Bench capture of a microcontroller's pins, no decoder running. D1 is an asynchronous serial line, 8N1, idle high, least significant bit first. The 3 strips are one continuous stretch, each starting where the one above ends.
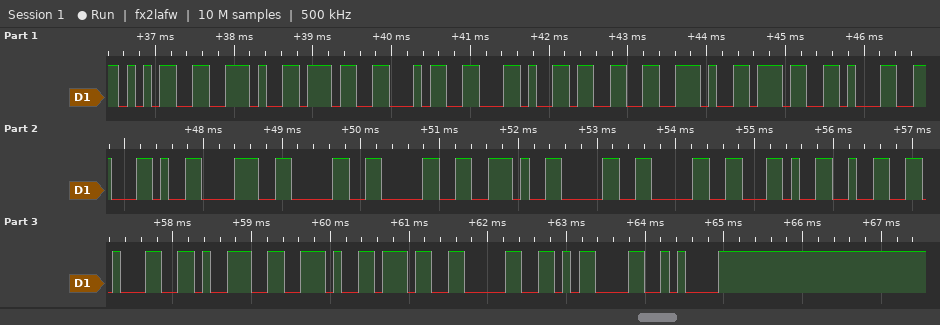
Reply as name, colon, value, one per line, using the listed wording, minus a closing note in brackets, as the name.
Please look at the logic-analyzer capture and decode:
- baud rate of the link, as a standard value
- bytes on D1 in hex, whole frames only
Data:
baud rate of the link, as a standard value: 9600 baud
bytes on D1 in hex, whole frames only: 0x35 0x2E 0x37 0x34 0x2C 0x33 0x2E 0x37 0x31 0x2C 0x38 0x30 0x30 0x2E 0x30 0x30 0x2C 0x32 0x31 0x39 0x2E 0x37 0x30 0x0D 0x0A
